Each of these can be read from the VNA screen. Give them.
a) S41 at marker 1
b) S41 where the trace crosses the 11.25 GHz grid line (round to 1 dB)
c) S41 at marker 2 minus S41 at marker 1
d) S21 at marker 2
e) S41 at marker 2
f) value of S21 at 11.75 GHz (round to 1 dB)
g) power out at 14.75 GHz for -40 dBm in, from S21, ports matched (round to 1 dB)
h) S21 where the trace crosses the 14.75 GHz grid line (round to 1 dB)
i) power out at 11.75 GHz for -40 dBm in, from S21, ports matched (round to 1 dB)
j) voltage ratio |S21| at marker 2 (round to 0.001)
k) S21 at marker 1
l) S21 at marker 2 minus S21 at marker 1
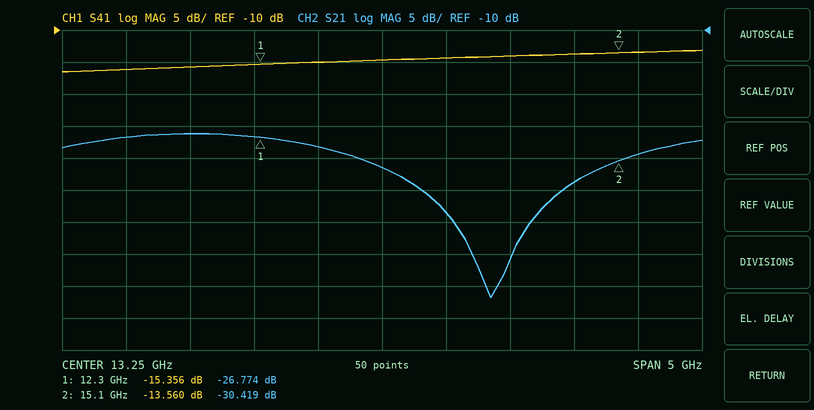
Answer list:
-15.356 dB
-16 dB
1.796 dB
-30.419 dB
-13.560 dB
-26 dB
-74 dBm
-34 dB
-66 dBm
0.030
-26.774 dB
-3.645 dB
